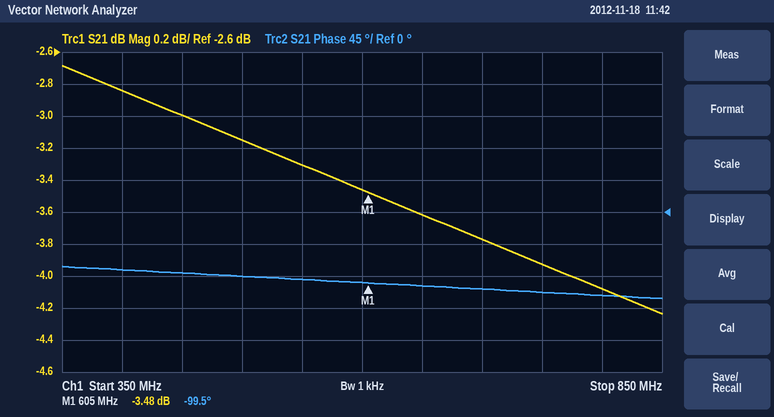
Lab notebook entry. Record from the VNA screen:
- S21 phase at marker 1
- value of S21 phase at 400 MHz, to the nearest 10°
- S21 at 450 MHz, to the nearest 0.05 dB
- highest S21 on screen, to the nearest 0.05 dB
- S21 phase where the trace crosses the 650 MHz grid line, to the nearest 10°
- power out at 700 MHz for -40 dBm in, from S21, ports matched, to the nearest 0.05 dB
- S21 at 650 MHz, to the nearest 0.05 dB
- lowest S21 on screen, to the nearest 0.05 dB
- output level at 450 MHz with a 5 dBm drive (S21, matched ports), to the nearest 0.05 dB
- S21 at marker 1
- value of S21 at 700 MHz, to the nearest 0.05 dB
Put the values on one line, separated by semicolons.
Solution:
-99.5°; -80°; -3.00 dB; -2.70 dB; -100°; -43.75 dBm; -3.60 dB; -4.25 dB; 2.00 dBm; -3.48 dB; -3.75 dB
